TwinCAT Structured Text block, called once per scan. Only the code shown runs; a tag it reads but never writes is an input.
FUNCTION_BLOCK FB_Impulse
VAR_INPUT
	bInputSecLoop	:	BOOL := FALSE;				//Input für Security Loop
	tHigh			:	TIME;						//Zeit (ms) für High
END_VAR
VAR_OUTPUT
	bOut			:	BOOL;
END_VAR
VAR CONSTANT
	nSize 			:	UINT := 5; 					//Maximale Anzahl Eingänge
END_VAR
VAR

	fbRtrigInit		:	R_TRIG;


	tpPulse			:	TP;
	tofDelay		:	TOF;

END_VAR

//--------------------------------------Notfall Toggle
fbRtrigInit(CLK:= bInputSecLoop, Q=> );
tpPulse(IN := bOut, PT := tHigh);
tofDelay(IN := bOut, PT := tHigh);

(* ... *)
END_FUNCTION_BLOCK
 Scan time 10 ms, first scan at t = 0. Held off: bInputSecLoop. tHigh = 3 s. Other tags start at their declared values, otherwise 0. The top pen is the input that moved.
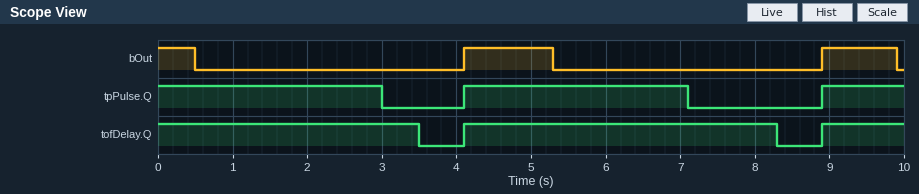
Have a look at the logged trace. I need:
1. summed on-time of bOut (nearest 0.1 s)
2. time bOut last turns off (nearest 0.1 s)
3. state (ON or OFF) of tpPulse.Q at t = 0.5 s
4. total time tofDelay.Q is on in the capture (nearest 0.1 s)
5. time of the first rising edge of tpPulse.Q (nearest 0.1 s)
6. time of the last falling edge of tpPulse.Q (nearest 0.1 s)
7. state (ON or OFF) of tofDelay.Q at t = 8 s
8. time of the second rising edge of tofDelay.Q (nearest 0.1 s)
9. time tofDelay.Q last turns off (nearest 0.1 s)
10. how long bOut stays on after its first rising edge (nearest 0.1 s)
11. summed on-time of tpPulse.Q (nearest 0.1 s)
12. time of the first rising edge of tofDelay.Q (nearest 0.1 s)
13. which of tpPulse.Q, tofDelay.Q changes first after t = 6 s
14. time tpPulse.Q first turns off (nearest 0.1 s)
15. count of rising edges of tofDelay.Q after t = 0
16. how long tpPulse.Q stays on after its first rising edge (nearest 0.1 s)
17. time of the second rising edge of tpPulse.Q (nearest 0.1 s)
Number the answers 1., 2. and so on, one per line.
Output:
1. 2.7 s
2. 9.9 s
3. ON
4. 8.8 s
5. 4.1 s
6. 7.1 s
7. ON
8. 8.9 s
9. 8.3 s
10. 1.2 s
11. 7.1 s
12. 4.1 s
13. tpPulse.Q
14. 3.0 s
15. 2
16. 3.0 s
17. 8.9 s
